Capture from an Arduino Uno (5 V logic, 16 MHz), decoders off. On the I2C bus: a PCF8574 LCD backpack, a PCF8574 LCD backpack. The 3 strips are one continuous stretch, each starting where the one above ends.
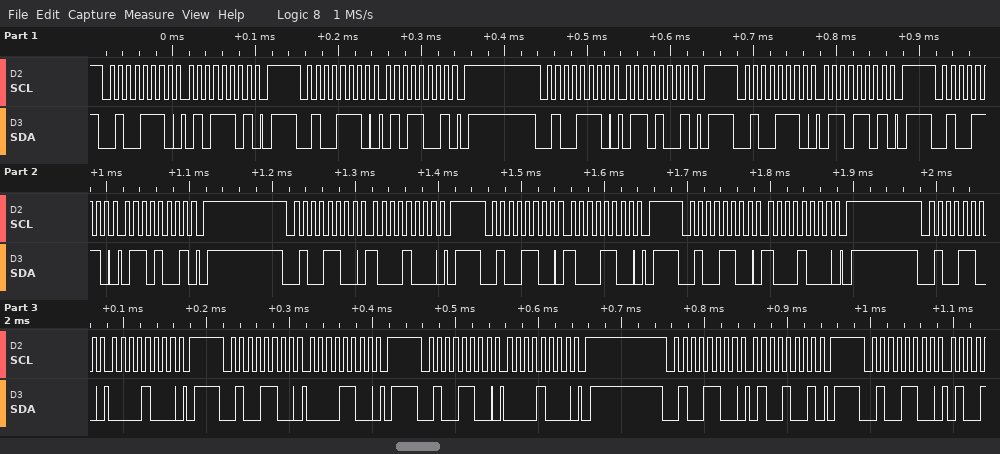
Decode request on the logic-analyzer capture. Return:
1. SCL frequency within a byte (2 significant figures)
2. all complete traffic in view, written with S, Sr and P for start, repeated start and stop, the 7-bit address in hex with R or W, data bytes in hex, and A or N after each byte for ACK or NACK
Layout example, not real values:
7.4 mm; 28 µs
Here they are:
100 kHz; S 27W A 5D A P S 27W A 59 A P S 27W A 69 A P S 27W A 6D A P S 27W A 69 A P S 26W A 88 A P S 26W A 8C A P S 26W A 88 A P S 26W A 08 A P S 26W A 0C A P S 26W A 08 A P S 26W A 49 A P S 26W A
